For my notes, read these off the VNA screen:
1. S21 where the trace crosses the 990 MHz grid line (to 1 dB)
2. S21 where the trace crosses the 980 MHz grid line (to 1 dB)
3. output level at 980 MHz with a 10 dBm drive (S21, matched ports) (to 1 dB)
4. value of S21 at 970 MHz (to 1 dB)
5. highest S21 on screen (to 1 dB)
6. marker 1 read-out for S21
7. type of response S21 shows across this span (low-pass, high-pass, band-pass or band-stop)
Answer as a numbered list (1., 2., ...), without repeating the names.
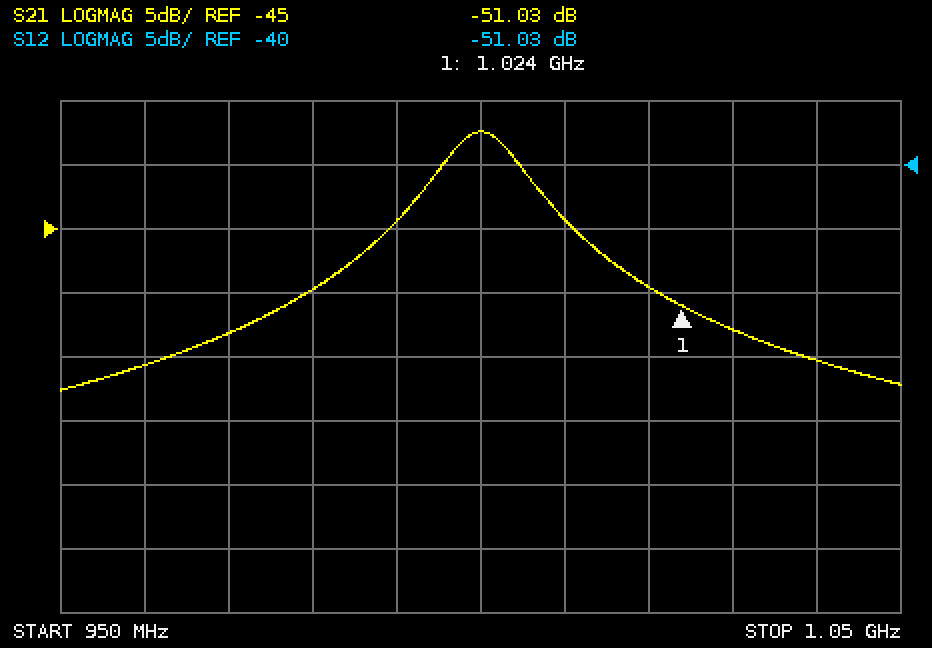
1. -44 dB
2. -50 dB
3. -40 dBm
4. -53 dB
5. -37 dB
6. -51.03 dB
7. band-pass
